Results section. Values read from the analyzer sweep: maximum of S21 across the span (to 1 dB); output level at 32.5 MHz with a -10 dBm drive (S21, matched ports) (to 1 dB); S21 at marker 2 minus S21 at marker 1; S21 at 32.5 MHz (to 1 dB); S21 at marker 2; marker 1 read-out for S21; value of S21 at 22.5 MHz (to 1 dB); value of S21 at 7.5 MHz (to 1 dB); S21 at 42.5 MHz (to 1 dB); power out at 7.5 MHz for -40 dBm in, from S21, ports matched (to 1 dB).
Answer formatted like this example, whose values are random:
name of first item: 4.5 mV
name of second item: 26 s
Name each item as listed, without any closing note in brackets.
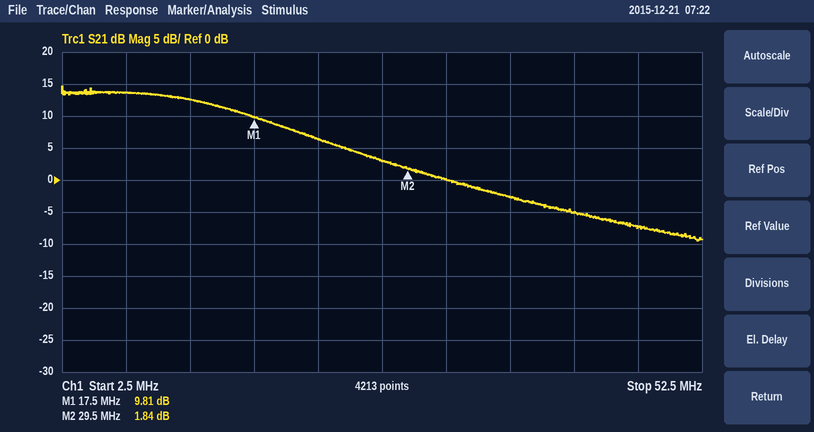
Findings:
maximum of S21 across the span: 15 dB
output level at 32.5 MHz with a -10 dBm drive (S21, matched ports): -10 dBm
S21 at marker 2 minus S21 at marker 1: -7.97 dB
S21 at 32.5 MHz: 0 dB
S21 at marker 2: 1.84 dB
marker 1 read-out for S21: 9.81 dB
value of S21 at 22.5 MHz: 6 dB
value of S21 at 7.5 MHz: 14 dB
S21 at 42.5 MHz: -5 dB
power out at 7.5 MHz for -40 dBm in, from S21, ports matched: -26 dBm
